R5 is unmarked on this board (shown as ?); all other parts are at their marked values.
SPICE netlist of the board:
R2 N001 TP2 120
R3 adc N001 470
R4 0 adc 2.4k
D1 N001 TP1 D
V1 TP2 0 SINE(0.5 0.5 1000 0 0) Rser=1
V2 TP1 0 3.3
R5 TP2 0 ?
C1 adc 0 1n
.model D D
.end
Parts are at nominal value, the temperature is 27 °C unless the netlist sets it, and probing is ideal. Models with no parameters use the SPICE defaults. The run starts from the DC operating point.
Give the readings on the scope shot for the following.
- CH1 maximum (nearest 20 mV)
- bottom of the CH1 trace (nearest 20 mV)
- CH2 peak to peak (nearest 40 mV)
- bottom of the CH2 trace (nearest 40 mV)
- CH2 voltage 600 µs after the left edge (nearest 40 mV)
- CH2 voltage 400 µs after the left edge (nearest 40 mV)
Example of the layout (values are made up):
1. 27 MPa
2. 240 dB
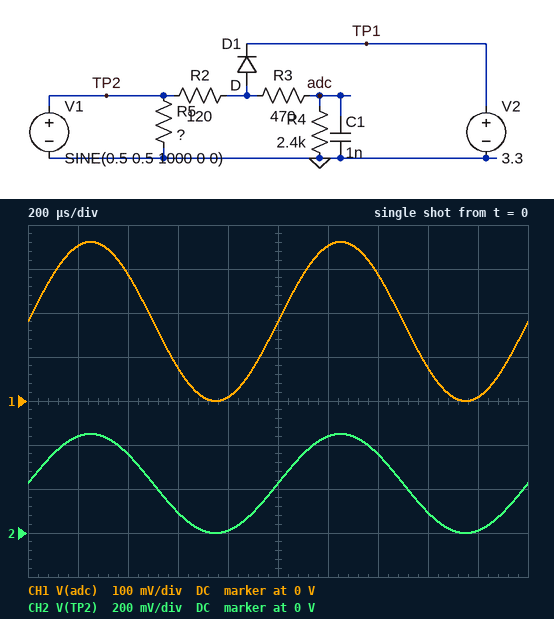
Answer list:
1. 360 mV
2. 0 V
3. 440 mV
4. 0 V
5. 80 mV
6. 360 mV
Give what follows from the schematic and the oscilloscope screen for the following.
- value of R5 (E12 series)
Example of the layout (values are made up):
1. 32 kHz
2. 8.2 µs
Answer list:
1. 0.82 Ω
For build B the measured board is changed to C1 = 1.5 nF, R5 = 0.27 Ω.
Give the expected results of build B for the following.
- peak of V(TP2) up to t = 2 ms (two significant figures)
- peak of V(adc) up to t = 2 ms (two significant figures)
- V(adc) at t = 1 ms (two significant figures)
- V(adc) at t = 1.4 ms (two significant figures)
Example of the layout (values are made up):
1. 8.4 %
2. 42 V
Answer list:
1. 210 mV
2. 170 mV
3. 85 mV
4. 140 mV
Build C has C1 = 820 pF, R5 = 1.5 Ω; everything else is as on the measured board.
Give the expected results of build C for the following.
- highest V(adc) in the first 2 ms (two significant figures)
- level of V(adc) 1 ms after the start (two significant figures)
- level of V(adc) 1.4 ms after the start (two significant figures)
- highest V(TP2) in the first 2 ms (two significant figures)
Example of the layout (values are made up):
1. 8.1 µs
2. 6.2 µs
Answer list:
1. 480 mV
2. 240 mV
3. 380 mV
4. 600 mV
